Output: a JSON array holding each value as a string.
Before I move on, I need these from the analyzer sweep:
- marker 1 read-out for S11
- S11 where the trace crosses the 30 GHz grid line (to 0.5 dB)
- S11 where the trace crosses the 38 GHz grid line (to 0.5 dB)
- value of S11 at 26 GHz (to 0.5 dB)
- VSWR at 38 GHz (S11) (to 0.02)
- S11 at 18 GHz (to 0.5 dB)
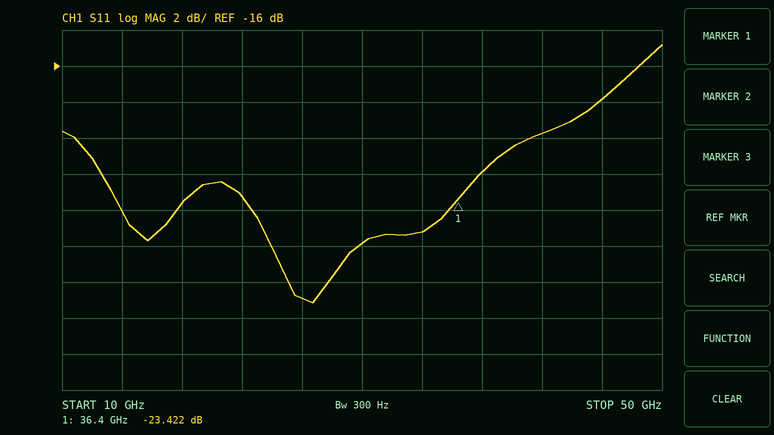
["-23.422 dB", "-26.0 dB", "-22.0 dB", "-29.0 dB", "1.18", "-23.5 dB"]
